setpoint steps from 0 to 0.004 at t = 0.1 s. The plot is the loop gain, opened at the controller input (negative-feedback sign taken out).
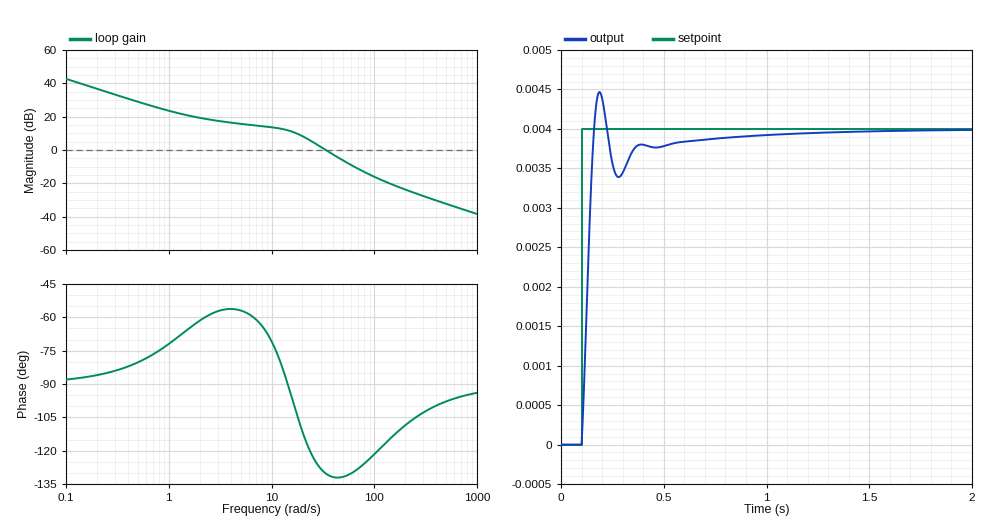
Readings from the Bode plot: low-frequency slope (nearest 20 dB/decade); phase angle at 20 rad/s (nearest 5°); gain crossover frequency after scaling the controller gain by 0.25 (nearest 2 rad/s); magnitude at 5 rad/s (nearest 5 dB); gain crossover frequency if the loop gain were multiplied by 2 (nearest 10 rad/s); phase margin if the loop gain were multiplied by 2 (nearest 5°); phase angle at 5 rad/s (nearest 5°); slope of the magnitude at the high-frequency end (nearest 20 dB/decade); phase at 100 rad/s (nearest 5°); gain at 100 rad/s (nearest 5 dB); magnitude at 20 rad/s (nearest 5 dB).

-20 dB/decade
-110°
14 rad/s
15 dB
50 rad/s
50°
-55°
-20 dB/decade
-120°
-15 dB
10 dB
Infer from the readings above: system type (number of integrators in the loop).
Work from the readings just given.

1
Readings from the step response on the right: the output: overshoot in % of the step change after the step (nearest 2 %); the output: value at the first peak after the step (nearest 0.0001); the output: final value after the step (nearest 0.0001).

12 %
0.0045
0.0040
